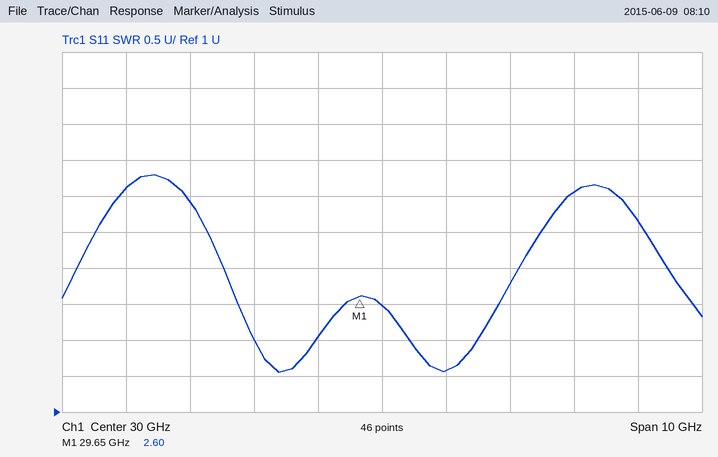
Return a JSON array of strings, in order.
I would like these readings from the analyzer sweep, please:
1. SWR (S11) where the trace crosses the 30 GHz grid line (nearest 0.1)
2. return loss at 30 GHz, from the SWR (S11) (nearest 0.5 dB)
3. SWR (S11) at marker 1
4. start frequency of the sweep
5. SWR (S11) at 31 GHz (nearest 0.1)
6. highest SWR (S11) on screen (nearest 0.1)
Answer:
["2.5", "7.5 dB", "2.60", "25 GHz", "1.6", "4.3"]
